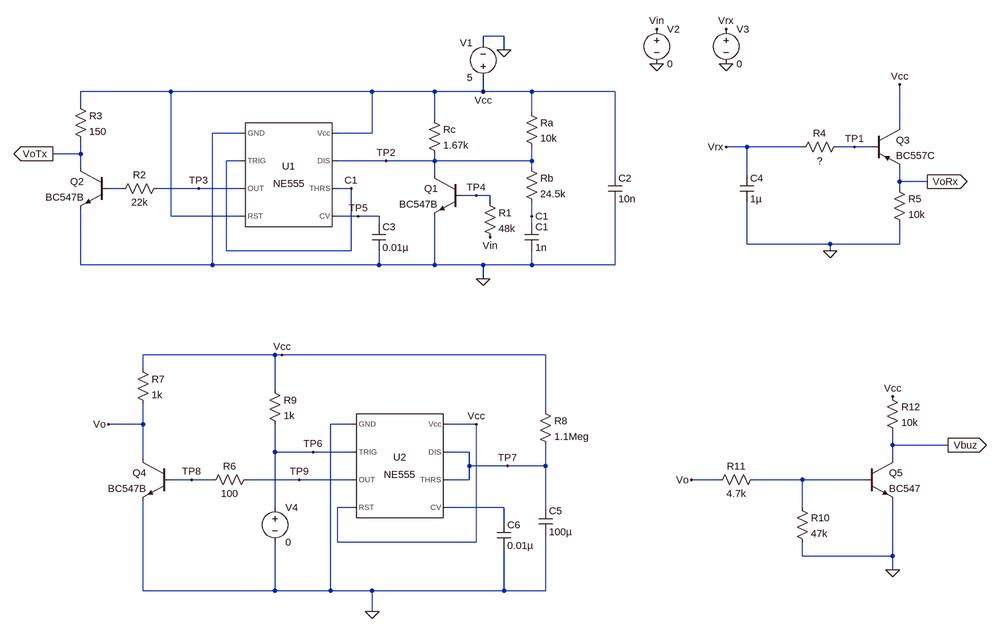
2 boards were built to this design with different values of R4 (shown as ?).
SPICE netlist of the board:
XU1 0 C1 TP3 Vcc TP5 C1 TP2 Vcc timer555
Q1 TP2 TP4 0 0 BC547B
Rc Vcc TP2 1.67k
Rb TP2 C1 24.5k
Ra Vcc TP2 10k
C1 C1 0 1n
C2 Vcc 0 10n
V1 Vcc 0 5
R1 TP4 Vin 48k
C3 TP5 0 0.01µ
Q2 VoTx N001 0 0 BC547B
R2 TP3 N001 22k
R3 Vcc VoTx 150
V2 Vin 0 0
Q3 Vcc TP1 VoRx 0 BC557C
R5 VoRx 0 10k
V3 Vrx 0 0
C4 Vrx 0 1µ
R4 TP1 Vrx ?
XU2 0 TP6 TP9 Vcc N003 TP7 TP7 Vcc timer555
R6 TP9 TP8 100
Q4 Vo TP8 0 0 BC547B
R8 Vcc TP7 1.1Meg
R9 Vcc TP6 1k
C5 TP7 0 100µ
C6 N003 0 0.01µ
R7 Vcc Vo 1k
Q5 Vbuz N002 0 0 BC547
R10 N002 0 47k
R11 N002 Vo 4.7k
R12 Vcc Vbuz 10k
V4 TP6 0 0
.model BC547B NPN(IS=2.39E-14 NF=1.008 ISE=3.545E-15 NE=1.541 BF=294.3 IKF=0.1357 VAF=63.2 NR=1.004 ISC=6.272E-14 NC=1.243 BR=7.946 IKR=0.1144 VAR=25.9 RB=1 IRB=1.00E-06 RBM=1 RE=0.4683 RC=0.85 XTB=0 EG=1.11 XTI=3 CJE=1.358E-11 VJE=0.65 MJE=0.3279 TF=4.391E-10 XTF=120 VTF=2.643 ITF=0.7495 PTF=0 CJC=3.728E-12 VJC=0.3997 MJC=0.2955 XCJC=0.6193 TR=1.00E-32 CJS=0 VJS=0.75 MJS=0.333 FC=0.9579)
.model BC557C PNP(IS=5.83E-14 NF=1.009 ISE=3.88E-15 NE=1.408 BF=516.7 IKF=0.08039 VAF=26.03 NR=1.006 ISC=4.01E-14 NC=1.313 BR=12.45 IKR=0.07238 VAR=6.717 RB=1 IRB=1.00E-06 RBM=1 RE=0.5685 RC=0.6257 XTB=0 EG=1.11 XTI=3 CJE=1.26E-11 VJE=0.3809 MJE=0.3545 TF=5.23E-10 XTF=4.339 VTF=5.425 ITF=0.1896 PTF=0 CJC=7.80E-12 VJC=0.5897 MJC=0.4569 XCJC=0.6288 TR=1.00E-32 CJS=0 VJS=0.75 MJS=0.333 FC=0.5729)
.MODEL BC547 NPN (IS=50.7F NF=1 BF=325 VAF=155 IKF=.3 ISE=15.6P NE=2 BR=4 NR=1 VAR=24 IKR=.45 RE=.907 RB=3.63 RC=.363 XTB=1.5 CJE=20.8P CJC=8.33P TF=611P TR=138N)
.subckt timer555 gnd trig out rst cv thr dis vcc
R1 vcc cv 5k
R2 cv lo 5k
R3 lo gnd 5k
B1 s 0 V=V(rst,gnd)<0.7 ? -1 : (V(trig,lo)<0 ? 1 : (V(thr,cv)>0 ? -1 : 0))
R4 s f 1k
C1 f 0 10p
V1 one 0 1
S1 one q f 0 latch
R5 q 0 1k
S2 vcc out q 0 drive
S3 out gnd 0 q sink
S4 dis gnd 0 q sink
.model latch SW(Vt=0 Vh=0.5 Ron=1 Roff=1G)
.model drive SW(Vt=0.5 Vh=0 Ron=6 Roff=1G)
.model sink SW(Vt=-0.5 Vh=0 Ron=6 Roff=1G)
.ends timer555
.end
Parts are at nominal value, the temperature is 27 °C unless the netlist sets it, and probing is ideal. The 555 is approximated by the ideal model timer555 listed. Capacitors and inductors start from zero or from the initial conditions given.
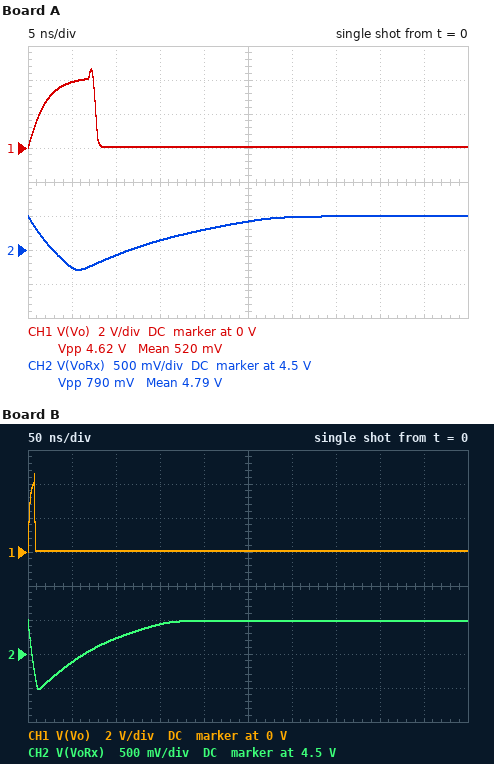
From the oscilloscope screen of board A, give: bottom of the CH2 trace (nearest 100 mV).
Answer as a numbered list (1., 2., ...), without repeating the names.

1. 4.2 V
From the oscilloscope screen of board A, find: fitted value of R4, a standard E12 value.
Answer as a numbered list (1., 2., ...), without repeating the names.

1. 5.6 kΩ
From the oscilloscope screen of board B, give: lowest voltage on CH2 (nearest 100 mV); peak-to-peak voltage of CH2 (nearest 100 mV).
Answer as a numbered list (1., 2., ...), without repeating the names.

1. 4.0 V
2. 1.0 V
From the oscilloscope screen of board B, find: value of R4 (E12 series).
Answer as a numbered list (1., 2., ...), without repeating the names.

1. 27 kΩ
